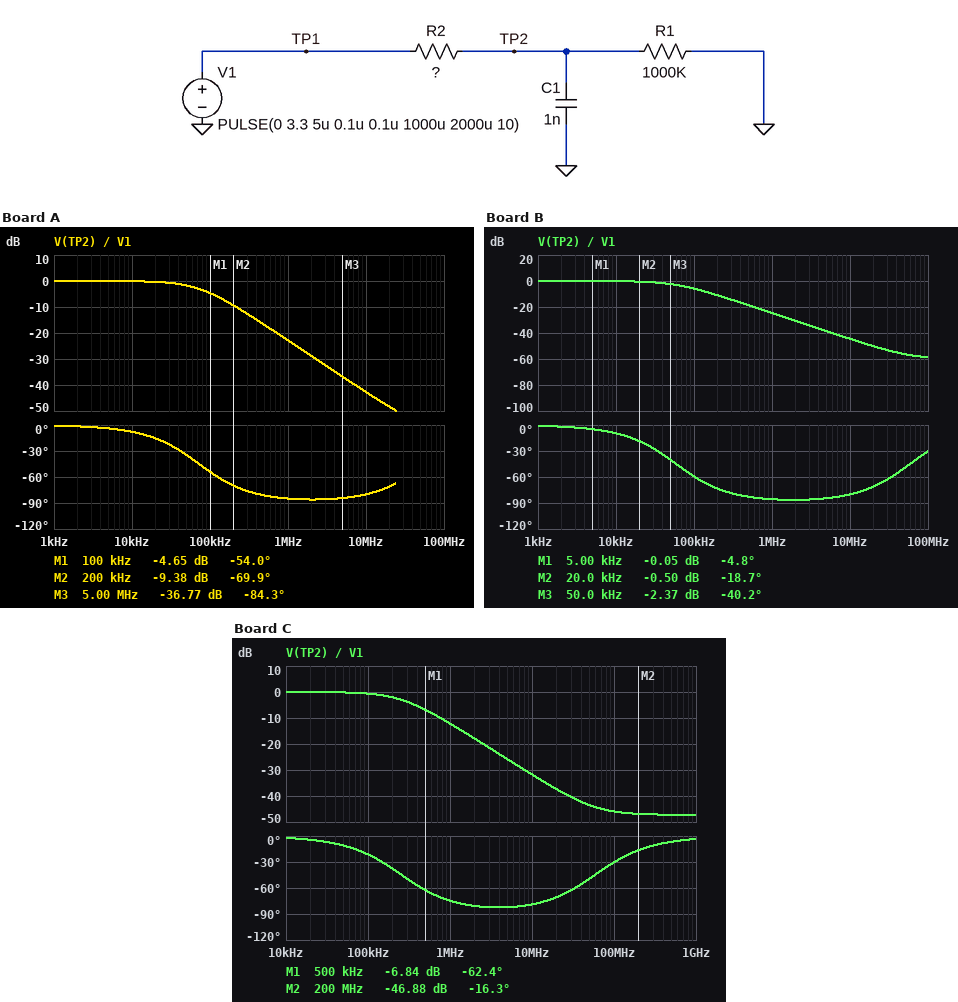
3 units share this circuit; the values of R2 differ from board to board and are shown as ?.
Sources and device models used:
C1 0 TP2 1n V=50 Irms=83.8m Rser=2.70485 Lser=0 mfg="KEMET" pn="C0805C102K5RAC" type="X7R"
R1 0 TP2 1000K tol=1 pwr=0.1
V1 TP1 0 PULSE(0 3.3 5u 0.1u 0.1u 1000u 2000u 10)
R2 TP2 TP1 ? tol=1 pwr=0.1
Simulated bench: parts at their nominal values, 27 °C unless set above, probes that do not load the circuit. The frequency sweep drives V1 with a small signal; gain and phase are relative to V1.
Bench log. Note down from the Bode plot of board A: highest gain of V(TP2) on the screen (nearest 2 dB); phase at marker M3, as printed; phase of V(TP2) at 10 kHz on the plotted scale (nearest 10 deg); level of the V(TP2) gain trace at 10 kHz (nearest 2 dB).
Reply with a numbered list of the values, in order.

1. 0 dB
2. -84.3 deg
3. -10 deg
4. 0 dB
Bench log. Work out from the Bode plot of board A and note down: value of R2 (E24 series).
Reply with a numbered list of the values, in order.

1. 2.2 kΩ
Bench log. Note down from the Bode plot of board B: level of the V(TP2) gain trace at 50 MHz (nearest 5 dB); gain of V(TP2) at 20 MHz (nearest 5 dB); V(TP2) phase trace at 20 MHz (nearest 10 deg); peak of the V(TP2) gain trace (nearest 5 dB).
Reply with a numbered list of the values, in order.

1. -55 dB
2. -50 dB
3. -70 deg
4. 0 dB
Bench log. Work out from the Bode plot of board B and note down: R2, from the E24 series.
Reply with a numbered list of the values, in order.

1. 2.7 kΩ
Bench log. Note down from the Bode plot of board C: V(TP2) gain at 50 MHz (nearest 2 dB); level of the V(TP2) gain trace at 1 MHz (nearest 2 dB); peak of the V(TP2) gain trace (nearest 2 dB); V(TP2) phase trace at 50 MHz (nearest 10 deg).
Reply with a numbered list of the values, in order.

1. -44 dB
2. -12 dB
3. 0 dB
4. -50 deg
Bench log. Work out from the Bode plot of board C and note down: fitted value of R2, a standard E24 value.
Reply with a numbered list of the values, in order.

1. 620 Ω
